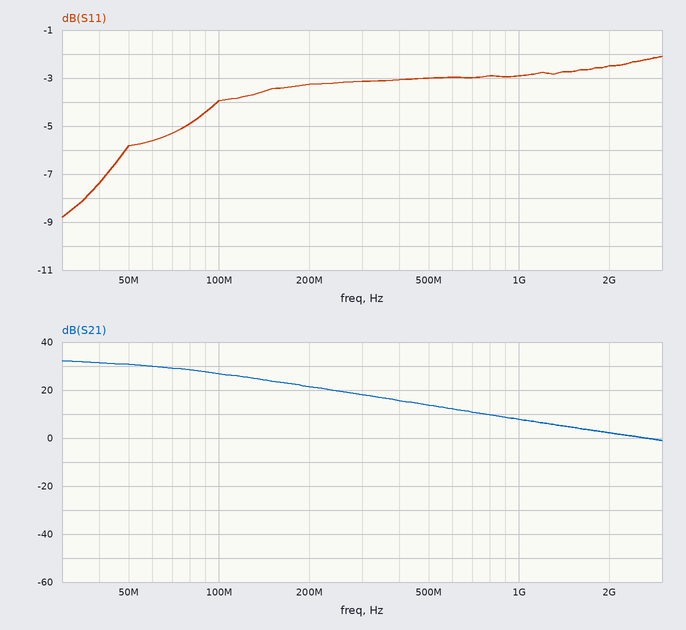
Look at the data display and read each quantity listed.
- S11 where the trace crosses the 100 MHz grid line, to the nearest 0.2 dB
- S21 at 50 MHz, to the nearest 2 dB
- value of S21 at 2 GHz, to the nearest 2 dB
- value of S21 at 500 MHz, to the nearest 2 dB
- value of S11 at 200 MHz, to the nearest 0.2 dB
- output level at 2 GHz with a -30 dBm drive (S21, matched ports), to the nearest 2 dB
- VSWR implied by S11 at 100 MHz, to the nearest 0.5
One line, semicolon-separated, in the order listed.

-4.0 dB; 30 dB; 2 dB; 14 dB; -3.2 dB; -28 dBm; 4.5
